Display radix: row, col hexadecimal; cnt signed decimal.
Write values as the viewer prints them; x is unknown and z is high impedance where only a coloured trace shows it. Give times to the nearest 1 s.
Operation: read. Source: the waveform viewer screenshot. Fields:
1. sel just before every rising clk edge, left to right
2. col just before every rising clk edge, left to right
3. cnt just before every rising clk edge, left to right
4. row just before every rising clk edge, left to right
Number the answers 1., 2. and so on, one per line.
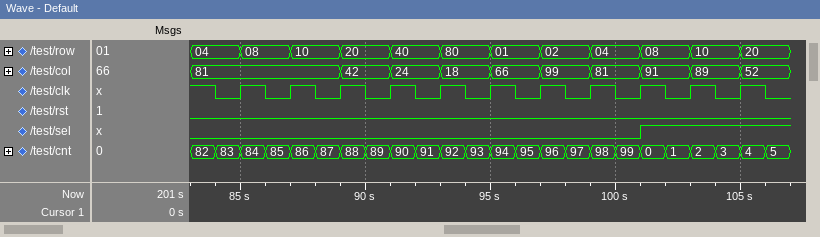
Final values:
1. 0 0 0 0 0 0 0 0 0 1 1
2. 81, 81, 81, 42, 24, 18, 66, 99, 81, 91, 89
3. 83, 85, 87, 89, 91, 93, 95, 97, 99, 1, 3
4. 04, 08, 10, 20, 40, 80, 01, 02, 04, 08, 10
